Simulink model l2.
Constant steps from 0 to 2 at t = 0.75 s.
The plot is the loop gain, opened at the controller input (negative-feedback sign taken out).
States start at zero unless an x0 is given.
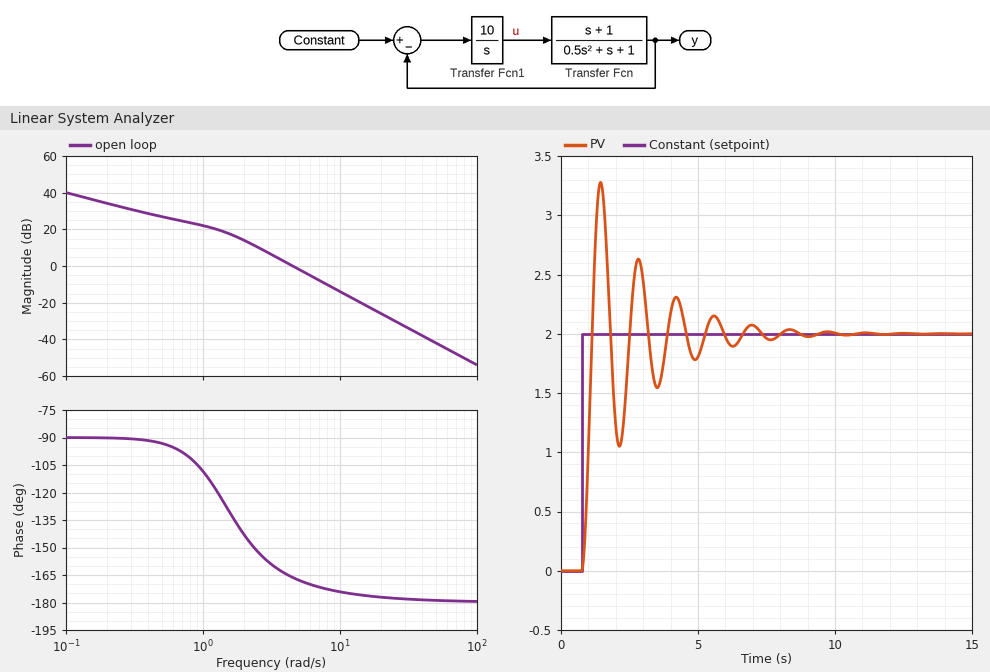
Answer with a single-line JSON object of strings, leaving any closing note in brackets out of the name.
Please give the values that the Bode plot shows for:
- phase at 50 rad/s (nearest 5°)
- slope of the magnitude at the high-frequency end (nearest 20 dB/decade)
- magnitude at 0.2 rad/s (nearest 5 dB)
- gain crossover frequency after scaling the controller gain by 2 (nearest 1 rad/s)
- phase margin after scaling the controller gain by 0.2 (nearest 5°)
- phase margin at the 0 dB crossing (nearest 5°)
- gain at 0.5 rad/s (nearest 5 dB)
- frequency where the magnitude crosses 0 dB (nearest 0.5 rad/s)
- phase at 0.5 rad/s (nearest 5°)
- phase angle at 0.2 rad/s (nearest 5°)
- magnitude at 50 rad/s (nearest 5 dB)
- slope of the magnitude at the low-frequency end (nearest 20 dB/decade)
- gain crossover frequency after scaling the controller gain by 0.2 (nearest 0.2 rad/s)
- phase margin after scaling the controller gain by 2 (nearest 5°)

{"phase at 50 rad/s": "-180°", "slope of the magnitude at the high-frequency end": "-40 dB/decade", "magnitude at 0.2 rad/s": "35 dB", "gain crossover frequency after scaling the controller gain by 2": "6 rad/s", "phase margin after scaling the controller gain by 0.2": "35°", "phase margin at the 0 dB crossing": "15°", "gain at 0.5 rad/s": "25 dB", "frequency where the magnitude crosses 0 dB": "4.5 rad/s", "phase at 0.5 rad/s": "-95°", "phase angle at 0.2 rad/s": "-90°", "magnitude at 50 rad/s": "-40 dB", "slope of the magnitude at the low-frequency end": "-20 dB/decade", "gain crossover frequency after scaling the controller gain by 0.2": "2.0 rad/s", "phase margin after scaling the controller gain by 2": "10°"}
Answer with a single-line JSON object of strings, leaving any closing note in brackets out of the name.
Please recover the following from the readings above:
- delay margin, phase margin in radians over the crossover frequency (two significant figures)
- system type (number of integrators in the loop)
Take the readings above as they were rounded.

{"delay margin, phase margin in radians over the crossover frequency": "0.058 s", "system type": "1"}
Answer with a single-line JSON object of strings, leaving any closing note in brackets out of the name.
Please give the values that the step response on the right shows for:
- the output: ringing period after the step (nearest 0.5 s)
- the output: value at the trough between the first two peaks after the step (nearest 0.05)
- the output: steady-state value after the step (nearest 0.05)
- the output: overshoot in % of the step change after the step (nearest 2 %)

{"the output: ringing period after the step": "1.5 s", "the output: value at the trough between the first two peaks after the step": "1.05", "the output: steady-state value after the step": "2.00", "the output: overshoot in % of the step change after the step": "64 %"}
